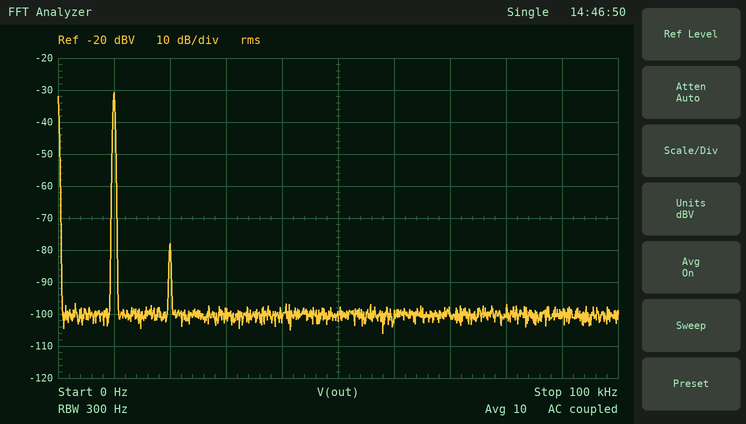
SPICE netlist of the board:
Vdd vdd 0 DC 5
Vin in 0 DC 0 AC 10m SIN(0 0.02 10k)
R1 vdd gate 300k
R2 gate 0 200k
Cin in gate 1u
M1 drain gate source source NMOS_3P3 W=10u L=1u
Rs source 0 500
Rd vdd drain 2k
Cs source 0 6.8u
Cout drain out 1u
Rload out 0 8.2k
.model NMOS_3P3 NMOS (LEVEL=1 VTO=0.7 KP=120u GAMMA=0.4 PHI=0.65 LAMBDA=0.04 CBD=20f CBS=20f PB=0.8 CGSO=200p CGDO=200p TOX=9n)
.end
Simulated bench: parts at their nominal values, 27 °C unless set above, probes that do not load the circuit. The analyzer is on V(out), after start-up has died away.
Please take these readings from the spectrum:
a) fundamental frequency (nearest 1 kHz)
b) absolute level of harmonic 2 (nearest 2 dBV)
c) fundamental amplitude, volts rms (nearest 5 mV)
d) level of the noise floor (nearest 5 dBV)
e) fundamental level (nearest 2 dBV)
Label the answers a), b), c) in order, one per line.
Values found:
a) 10 kHz
b) -78 dBV
c) 30 mV
d) -100 dBV
e) -30 dBV
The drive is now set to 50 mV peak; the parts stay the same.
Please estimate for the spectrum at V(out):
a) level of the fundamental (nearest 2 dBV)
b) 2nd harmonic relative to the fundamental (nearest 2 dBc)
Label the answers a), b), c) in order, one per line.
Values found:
a) -22 dBV
b) -40 dBc
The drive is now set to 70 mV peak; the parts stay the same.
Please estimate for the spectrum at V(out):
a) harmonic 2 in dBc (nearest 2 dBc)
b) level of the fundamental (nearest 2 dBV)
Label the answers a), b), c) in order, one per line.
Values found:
a) -36 dBc
b) -20 dBV
